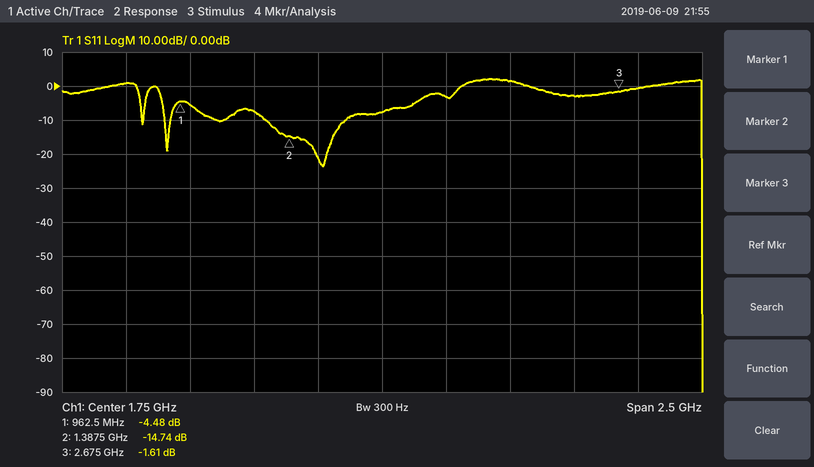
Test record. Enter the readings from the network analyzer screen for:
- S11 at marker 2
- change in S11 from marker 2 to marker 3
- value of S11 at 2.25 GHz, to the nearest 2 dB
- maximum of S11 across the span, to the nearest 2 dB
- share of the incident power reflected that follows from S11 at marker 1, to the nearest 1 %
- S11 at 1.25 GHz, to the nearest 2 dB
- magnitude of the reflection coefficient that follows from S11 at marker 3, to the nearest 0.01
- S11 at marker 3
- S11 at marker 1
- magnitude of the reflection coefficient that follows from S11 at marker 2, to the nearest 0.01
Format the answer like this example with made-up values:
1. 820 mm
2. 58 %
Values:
1. -14.74 dB
2. 13.13 dB
3. 2 dB
4. 2 dB
5. 36 %
6. -8 dB
7. 0.83
8. -1.61 dB
9. -4.48 dB
10. 0.18
